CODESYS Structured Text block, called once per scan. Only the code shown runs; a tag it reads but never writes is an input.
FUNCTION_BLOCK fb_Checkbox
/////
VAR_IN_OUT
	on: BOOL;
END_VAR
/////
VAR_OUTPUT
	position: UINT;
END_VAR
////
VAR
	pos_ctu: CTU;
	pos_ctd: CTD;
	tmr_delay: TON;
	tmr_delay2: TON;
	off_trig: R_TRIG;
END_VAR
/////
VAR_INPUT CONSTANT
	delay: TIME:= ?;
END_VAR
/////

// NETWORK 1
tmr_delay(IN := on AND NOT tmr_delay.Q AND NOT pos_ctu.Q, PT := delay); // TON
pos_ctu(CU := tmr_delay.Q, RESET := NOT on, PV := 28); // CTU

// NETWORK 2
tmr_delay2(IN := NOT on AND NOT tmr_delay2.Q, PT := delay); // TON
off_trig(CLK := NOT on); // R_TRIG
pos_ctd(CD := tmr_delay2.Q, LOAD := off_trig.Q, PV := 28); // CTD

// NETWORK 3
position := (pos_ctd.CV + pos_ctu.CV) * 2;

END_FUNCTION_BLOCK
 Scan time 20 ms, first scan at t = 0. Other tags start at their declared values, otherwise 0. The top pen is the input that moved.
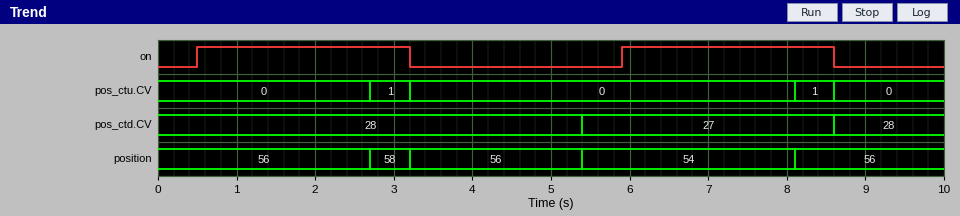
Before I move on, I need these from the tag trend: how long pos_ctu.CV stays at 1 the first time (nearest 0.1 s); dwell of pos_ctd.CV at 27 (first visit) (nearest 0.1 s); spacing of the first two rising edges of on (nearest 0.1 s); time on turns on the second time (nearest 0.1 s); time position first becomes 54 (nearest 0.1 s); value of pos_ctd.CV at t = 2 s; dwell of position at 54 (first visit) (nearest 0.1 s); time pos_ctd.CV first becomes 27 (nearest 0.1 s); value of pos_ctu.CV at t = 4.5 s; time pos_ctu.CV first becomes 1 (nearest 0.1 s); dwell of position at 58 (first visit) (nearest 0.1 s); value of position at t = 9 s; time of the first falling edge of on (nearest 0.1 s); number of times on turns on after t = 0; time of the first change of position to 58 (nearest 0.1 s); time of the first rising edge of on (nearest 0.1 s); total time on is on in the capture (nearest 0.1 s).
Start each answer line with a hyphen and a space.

- 0.5 s
- 3.2 s
- 5.4 s
- 5.9 s
- 5.4 s
- 28
- 2.7 s
- 5.4 s
- 0
- 2.7 s
- 0.5 s
- 56
- 3.2 s
- 2
- 2.7 s
- 0.5 s
- 5.4 s
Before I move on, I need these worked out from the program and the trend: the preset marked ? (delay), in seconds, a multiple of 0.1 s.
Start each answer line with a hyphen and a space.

- 2.2 s
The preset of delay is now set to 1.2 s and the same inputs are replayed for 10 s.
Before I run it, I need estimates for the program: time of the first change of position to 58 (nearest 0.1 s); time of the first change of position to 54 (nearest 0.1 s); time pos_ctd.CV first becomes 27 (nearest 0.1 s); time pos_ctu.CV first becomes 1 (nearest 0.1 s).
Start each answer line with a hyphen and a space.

- 1.7 s
- 4.4 s
- 4.4 s
- 1.7 s
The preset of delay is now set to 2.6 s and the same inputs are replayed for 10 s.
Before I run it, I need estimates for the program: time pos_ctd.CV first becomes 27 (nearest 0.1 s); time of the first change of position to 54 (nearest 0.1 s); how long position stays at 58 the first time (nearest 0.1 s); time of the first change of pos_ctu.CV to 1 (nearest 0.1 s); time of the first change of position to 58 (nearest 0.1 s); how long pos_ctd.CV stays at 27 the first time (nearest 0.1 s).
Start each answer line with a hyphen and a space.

- 5.8 s
- 5.8 s
- 0.1 s
- 3.1 s
- 3.1 s
- 2.8 s
